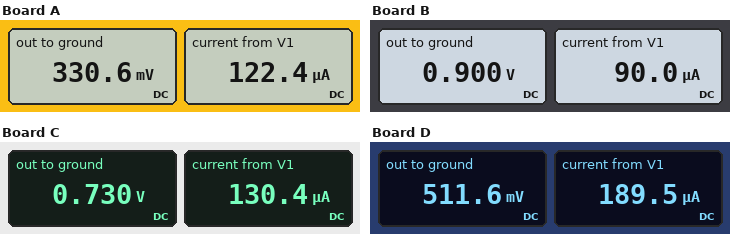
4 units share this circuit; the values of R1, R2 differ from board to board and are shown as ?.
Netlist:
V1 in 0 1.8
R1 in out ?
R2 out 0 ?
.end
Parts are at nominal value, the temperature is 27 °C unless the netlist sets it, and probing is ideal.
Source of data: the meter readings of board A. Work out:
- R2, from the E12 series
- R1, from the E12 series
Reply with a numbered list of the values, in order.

1. 2.7 kΩ
2. 12 kΩ
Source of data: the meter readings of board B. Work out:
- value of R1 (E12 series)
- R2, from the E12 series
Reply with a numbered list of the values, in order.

1. 10 kΩ
2. 10 kΩ
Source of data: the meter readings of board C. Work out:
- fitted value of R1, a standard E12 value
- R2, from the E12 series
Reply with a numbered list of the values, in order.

1. 8.2 kΩ
2. 5.6 kΩ
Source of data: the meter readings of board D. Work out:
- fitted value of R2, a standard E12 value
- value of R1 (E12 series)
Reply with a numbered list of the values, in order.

1. 2.7 kΩ
2. 6.8 kΩ
